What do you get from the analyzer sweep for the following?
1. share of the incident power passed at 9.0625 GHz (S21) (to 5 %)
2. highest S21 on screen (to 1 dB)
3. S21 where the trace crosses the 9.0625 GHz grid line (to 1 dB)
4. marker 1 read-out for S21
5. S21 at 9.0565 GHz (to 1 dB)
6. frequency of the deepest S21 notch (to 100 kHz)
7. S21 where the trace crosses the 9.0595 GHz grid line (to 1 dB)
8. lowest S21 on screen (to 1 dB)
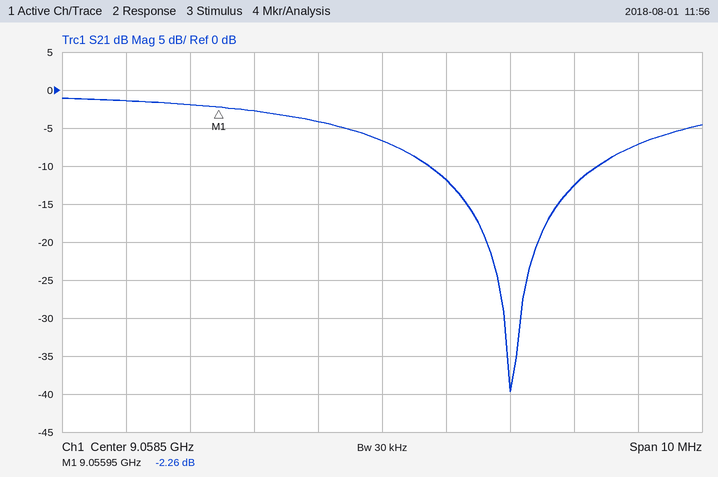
20 %
-1 dB
-7 dB
-2.26 dB
-3 dB
9.0605 GHz
-12 dB
-40 dB
